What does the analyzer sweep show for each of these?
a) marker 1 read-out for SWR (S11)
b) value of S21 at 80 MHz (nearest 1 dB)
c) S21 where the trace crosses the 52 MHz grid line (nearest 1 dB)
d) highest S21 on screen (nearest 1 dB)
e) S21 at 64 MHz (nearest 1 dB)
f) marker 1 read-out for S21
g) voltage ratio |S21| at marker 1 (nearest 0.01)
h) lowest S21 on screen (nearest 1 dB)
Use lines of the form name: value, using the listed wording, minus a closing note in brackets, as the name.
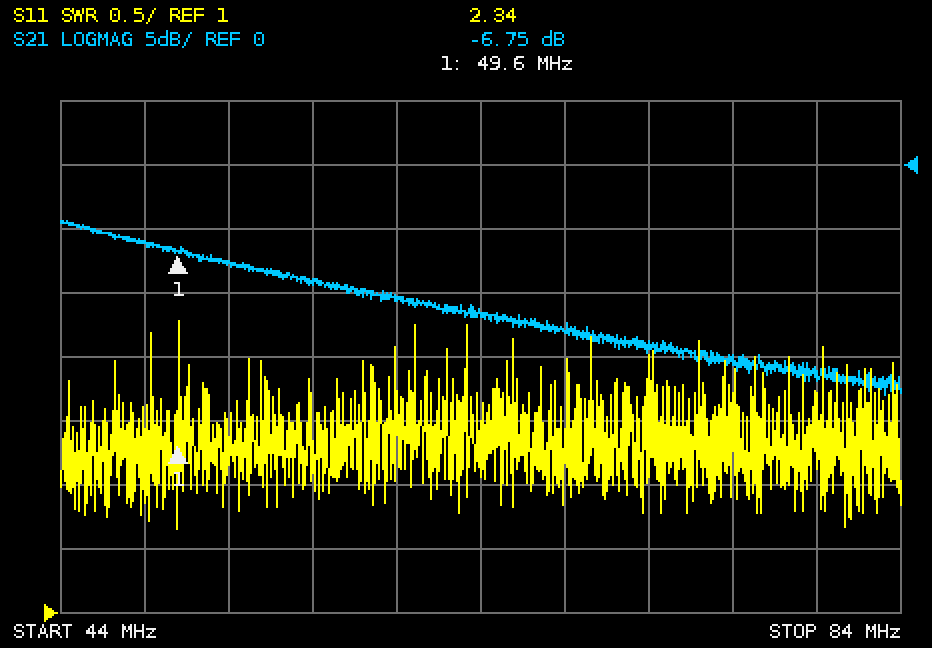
marker 1 read-out for SWR: 2.34
value of S21 at 80 MHz: -16 dB
S21 where the trace crosses the 52 MHz grid line: -8 dB
highest S21 on screen: -4 dB
S21 at 64 MHz: -12 dB
marker 1 read-out for S21: -6.75 dB
voltage ratio |S21| at marker 1: 0.46
lowest S21 on screen: -18 dB
